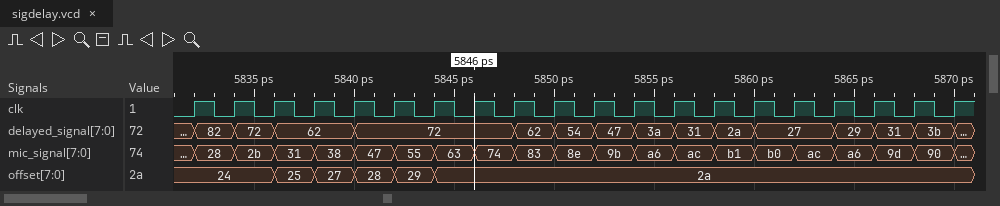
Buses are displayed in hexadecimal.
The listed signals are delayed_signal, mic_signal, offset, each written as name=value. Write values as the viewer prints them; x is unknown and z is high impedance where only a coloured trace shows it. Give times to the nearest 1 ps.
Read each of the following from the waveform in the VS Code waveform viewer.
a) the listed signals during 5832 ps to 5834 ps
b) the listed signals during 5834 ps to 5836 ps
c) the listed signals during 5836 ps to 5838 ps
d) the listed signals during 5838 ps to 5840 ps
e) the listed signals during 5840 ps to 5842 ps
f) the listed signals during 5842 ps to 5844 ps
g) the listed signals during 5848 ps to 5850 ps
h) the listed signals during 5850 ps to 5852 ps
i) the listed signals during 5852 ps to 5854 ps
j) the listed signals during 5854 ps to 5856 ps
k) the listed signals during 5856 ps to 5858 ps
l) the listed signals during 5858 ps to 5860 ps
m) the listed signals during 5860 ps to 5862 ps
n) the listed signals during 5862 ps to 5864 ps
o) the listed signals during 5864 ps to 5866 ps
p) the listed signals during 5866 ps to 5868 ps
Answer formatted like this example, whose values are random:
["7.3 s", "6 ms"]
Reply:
["delayed_signal=82, mic_signal=28, offset=24", "delayed_signal=72, mic_signal=2b, offset=24", "delayed_signal=62, mic_signal=31, offset=25", "delayed_signal=62, mic_signal=38, offset=27", "delayed_signal=72, mic_signal=47, offset=28", "delayed_signal=72, mic_signal=55, offset=29", "delayed_signal=62, mic_signal=83, offset=2a", "delayed_signal=54, mic_signal=8e, offset=2a", "delayed_signal=47, mic_signal=9b, offset=2a", "delayed_signal=3a, mic_signal=a6, offset=2a", "delayed_signal=31, mic_signal=ac, offset=2a", "delayed_signal=2a, mic_signal=b1, offset=2a", "delayed_signal=27, mic_signal=b0, offset=2a", "delayed_signal=27, mic_signal=ac, offset=2a", "delayed_signal=29, mic_signal=a6, offset=2a", "delayed_signal=31, mic_signal=9d, offset=2a"]
